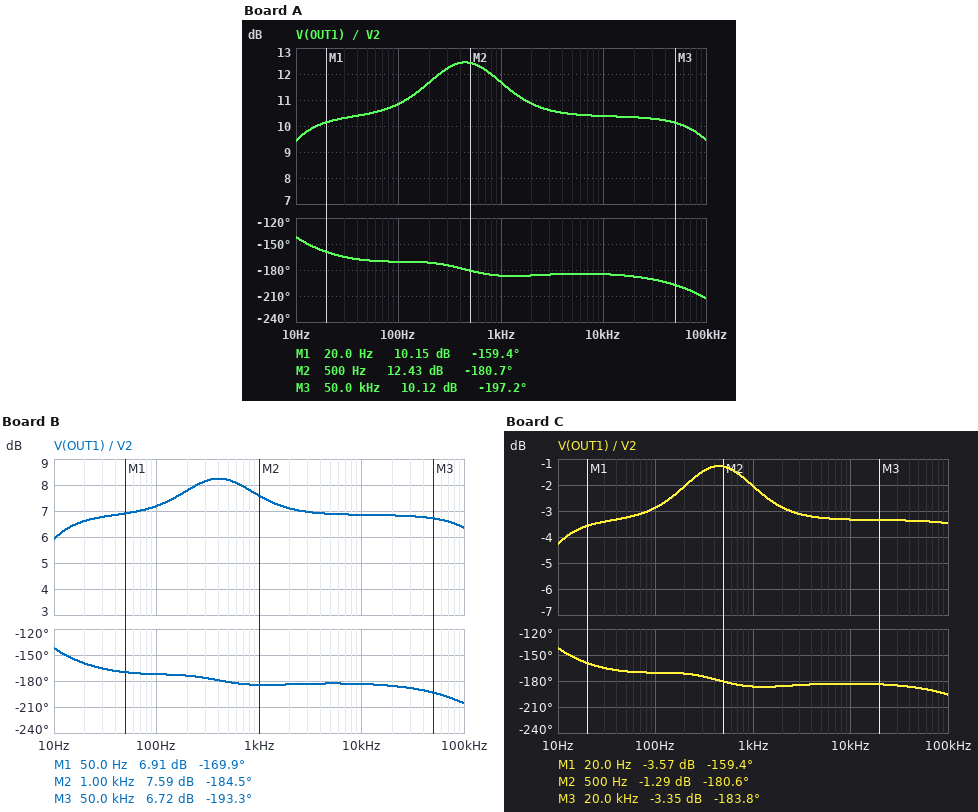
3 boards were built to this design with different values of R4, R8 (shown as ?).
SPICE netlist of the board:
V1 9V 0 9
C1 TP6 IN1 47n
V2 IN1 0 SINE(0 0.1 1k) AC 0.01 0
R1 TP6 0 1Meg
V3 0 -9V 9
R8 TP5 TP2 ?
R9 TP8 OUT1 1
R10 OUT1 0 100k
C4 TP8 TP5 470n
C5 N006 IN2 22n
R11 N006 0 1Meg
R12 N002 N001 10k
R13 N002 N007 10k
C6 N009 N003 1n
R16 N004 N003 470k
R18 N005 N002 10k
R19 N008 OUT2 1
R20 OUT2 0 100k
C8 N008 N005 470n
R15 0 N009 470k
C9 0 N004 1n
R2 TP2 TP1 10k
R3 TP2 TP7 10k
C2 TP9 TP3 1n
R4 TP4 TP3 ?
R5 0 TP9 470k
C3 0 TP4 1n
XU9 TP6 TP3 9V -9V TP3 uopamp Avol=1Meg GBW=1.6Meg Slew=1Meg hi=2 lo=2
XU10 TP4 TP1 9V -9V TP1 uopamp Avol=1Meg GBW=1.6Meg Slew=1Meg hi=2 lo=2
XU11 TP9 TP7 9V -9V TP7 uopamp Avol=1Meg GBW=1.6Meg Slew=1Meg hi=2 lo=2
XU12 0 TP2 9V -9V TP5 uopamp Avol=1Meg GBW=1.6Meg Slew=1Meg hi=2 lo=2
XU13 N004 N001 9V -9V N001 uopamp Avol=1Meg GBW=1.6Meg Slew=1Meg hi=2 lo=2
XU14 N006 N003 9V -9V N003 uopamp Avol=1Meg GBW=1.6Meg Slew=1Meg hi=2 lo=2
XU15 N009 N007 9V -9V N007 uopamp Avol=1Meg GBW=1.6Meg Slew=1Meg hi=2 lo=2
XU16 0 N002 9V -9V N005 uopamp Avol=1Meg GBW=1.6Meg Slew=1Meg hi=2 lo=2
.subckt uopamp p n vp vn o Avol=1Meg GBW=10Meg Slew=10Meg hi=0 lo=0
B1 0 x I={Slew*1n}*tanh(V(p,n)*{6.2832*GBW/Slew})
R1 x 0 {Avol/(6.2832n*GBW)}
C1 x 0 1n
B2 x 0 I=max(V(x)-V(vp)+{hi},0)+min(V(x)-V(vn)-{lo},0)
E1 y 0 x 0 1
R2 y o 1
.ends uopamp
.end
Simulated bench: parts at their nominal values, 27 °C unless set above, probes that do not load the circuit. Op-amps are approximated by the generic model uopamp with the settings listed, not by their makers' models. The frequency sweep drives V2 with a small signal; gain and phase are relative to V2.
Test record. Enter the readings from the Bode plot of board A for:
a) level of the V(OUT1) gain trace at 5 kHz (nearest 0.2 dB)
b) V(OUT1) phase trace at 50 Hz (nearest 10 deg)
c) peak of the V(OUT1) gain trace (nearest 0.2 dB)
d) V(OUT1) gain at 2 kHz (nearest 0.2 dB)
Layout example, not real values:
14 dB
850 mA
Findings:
10.4 dB
-170 deg
12.4 dB
10.8 dB
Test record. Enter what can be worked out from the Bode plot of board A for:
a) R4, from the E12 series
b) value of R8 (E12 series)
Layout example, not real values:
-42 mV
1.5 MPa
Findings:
270 kΩ
33 kΩ
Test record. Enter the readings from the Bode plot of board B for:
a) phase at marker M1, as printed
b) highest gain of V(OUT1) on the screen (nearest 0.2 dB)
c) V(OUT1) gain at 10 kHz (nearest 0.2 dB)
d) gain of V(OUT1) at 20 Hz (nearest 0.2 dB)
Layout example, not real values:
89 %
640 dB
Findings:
-169.9 deg
8.2 dB
6.8 dB
6.6 dB
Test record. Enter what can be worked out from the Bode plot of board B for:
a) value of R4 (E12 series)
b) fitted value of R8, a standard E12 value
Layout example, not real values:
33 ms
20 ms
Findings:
330 kΩ
22 kΩ
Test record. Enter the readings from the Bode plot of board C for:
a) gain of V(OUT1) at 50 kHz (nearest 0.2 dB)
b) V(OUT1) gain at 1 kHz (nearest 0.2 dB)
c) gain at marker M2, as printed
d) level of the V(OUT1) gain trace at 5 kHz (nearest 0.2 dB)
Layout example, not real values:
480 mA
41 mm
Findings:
-3.4 dB
-2.0 dB
-1.29 dB
-3.2 dB
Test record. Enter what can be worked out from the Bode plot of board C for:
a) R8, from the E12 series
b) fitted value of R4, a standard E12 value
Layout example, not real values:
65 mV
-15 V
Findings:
6.8 kΩ
270 kΩ
